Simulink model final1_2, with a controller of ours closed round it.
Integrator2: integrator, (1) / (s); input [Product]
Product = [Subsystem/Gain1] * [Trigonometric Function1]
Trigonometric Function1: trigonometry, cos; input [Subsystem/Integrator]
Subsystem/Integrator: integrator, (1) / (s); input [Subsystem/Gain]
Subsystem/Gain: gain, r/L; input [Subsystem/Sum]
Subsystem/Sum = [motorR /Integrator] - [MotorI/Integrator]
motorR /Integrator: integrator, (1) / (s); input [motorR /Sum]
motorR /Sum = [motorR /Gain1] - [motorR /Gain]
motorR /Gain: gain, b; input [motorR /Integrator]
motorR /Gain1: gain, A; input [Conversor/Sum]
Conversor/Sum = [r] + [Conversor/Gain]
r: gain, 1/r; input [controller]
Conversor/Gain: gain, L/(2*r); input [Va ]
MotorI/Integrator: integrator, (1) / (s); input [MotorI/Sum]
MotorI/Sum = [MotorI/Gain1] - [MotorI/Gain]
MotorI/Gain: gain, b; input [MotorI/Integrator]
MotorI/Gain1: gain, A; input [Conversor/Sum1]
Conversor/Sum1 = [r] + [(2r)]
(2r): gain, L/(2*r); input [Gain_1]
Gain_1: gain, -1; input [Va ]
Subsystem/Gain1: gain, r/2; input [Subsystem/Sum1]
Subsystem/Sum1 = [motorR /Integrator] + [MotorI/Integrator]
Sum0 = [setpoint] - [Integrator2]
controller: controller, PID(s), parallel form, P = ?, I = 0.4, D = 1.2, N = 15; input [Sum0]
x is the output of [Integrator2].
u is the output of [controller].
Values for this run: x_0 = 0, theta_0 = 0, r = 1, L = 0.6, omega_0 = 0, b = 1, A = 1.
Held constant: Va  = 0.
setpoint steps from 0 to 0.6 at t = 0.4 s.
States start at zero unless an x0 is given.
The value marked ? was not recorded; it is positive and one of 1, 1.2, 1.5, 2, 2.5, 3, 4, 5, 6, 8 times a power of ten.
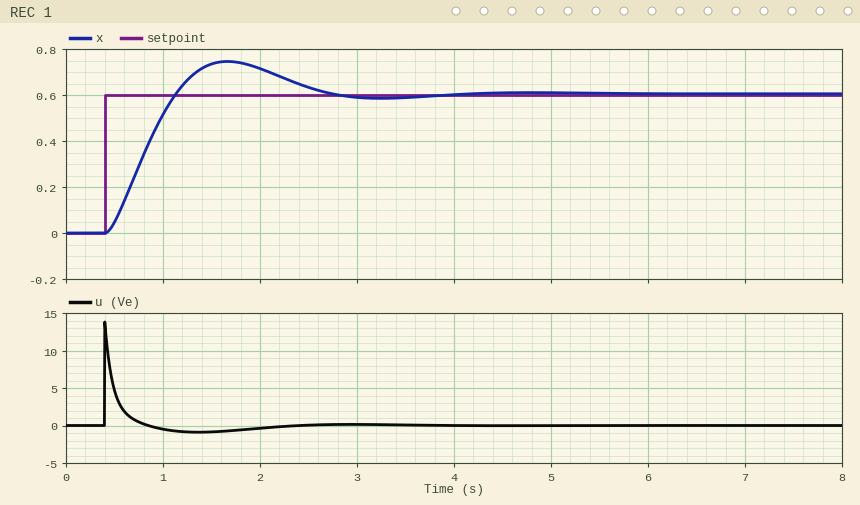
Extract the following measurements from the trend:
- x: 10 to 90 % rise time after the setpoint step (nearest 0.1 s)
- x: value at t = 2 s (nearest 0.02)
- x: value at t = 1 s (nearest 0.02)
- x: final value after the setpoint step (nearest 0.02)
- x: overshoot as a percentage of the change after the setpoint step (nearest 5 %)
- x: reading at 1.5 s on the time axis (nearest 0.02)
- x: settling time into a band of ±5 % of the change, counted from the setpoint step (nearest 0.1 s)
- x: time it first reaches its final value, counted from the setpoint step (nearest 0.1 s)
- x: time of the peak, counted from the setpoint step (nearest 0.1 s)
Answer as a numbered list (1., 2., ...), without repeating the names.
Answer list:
1. 0.5 s
2. 0.72
3. 0.52
4. 0.60
5. 25 %
6. 0.74
7. 2.1 s
8. 0.7 s
9. 1.3 s
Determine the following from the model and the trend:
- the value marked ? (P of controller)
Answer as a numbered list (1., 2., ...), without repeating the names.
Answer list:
1. 5
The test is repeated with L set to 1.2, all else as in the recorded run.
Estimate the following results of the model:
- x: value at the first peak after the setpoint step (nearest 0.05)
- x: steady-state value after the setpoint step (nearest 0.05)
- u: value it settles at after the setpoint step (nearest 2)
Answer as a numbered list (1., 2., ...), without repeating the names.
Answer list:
1. 0.75
2. 0.60
3. 0
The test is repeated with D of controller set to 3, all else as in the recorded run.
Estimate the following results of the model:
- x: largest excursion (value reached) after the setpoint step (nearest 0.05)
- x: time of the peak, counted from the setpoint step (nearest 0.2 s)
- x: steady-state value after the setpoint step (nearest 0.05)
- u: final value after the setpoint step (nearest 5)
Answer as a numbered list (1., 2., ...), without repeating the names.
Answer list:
1. 0.65
2. 1.0 s
3. 0.60
4. 0
